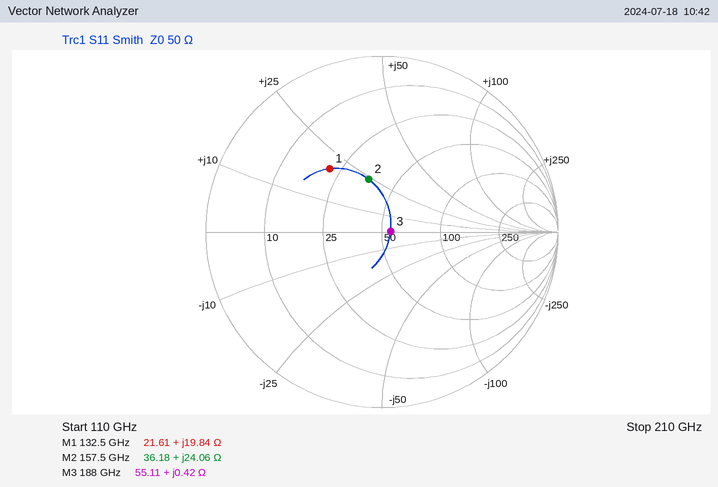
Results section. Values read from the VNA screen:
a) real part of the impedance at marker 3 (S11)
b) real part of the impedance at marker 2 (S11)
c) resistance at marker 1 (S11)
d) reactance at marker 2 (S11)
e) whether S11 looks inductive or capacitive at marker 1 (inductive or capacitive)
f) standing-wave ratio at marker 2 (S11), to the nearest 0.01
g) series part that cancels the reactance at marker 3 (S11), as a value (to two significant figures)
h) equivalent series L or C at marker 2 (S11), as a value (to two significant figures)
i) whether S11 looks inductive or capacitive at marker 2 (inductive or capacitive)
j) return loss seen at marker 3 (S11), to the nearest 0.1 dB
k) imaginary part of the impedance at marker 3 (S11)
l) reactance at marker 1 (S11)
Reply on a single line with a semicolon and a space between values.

55.11 Ω; 36.18 Ω; 21.61 Ω; +24.06 Ω; inductive; 1.90; 2.0 pF; 24 pH; inductive; 26.2 dB; +0.42 Ω; +19.84 Ω
